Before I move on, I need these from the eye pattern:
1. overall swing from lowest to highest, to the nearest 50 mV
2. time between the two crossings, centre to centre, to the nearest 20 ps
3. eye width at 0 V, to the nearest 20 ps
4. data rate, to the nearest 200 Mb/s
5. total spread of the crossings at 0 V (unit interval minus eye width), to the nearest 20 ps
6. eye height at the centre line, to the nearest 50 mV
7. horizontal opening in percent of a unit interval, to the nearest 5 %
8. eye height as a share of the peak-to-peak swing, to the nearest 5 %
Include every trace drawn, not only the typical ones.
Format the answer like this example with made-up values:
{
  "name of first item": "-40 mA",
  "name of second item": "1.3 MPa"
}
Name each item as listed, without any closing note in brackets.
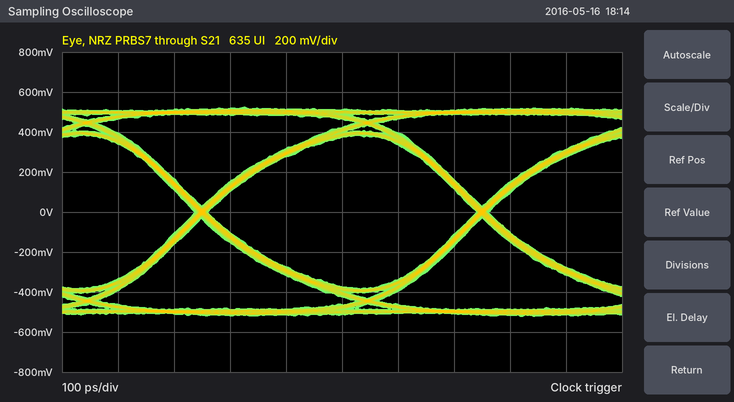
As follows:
{
  "overall swing from lowest to highest, to the nearest 50 mV": "1.05 V",
  "time between the two crossings, centre to centre, to the nearest 20 ps": "500 ps",
  "eye width at 0 V, to the nearest 20 ps": "480 ps",
  "data rate, to the nearest 200 Mb/s": "2.0 Gb/s",
  "total spread of the crossings at 0 V (unit interval minus eye width), to the nearest 20 ps": "20 ps",
  "eye height at the centre line, to the nearest 50 mV": "750 mV",
  "horizontal opening in percent of a unit interval, to the nearest 5 %": "95 %",
  "eye height as a share of the peak-to-peak swing, to the nearest 5 %": "70 %"
}
